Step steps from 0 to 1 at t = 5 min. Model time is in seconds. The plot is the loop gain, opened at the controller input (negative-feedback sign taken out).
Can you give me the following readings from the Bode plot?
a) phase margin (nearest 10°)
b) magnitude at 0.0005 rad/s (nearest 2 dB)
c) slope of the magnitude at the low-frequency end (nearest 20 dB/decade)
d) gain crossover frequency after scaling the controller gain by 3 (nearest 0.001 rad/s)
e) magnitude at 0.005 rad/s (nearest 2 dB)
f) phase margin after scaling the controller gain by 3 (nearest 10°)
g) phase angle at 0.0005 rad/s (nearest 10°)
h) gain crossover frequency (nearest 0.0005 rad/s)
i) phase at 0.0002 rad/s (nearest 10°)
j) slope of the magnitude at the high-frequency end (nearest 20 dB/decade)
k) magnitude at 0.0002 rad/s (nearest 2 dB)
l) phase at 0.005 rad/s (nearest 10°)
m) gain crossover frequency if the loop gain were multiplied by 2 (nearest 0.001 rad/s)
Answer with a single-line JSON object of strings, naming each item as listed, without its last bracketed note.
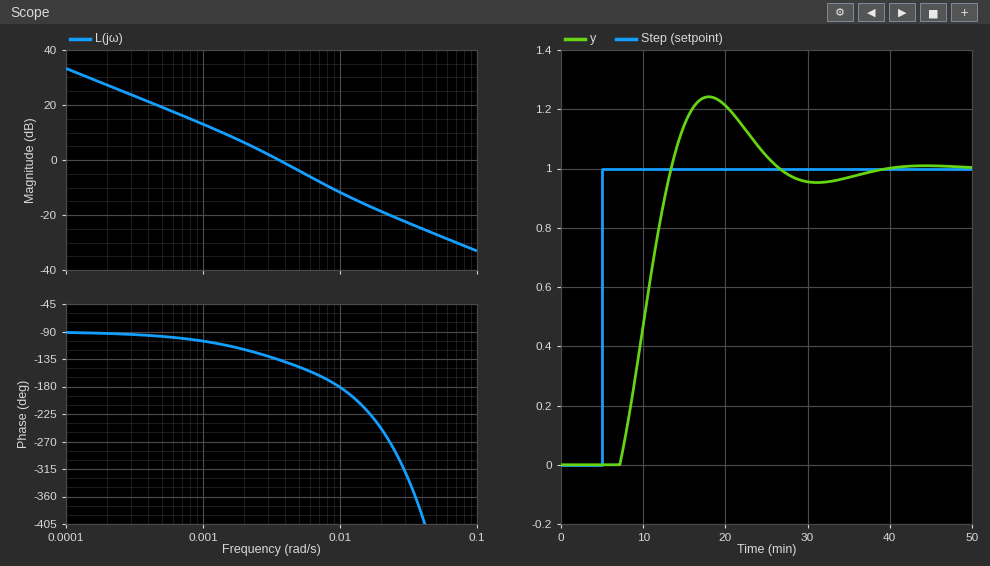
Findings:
{"phase margin": "40°", "magnitude at 0.0005 rad/s": "20 dB", "slope of the magnitude at the low-frequency end": "-20 dB/decade", "gain crossover frequency after scaling the controller gain by 3": "0.008 rad/s", "magnitude at 0.005 rad/s": "-4 dB", "phase margin after scaling the controller gain by 3": "10°", "phase angle at 0.0005 rad/s": "-100°", "gain crossover frequency": "0.0035 rad/s", "phase at 0.0002 rad/s": "-90°", "slope of the magnitude at the high-frequency end": "-20 dB/decade", "magnitude at 0.0002 rad/s": "28 dB", "phase at 0.005 rad/s": "-150°", "gain crossover frequency if the loop gain were multiplied by 2": "0.006 rad/s"}
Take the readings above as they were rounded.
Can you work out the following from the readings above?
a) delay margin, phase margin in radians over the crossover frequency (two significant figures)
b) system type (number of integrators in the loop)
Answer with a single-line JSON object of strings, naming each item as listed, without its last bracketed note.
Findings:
{"delay margin, phase margin in radians over the crossover frequency": "200 s", "system type": "1"}
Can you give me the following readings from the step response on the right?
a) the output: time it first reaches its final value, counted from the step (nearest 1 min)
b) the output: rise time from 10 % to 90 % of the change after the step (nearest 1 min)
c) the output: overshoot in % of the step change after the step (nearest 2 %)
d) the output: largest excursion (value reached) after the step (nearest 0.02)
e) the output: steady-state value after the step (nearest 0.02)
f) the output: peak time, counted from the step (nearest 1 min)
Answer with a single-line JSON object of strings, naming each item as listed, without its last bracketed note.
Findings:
{"the output: time it first reaches its final value, counted from the step": "8 min", "the output: rise time from 10 % to 90 % of the change after the step": "5 min", "the output: overshoot in % of the step change after the step": "24 %", "the output: largest excursion (value reached) after the step": "1.24", "the output: steady-state value after the step": "1.00", "the output: peak time, counted from the step": "13 min"}
